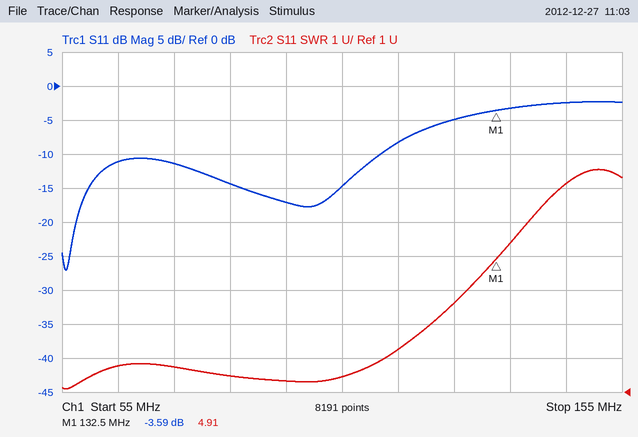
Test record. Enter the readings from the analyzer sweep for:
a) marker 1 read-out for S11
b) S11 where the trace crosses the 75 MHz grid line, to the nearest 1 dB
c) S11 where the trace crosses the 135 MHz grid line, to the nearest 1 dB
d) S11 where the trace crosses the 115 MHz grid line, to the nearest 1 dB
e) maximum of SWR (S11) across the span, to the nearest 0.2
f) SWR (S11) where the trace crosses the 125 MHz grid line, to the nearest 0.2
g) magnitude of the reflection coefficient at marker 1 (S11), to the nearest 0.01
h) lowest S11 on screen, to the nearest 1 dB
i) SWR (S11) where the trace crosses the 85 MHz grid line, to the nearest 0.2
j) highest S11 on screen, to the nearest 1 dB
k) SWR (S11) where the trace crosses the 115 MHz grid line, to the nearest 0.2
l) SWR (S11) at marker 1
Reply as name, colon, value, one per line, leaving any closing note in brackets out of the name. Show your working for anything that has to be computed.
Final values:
marker 1 read-out for S11: -3.59 dB
S11 where the trace crosses the 75 MHz grid line, to the nearest 1 dB: -11 dB
S11 where the trace crosses the 135 MHz grid line, to the nearest 1 dB: -3 dB
S11 where the trace crosses the 115 MHz grid line, to the nearest 1 dB: -8 dB
maximum of SWR (S11) across the span, to the nearest 0.2: 7.6
SWR (S11) where the trace crosses the 125 MHz grid line, to the nearest 0.2: 3.6
magnitude of the reflection coefficient at marker 1 (S11), to the nearest 0.01: 10^(-3.59/20) ≈ 0.66
lowest S11 on screen, to the nearest 1 dB: -27 dB
SWR (S11) where the trace crosses the 85 MHz grid line, to the nearest 0.2: 1.4
highest S11 on screen, to the nearest 1 dB: -2 dB
SWR (S11) where the trace crosses the 115 MHz grid line, to the nearest 0.2: 2.2
SWR (S11) at marker 1: 4.91
